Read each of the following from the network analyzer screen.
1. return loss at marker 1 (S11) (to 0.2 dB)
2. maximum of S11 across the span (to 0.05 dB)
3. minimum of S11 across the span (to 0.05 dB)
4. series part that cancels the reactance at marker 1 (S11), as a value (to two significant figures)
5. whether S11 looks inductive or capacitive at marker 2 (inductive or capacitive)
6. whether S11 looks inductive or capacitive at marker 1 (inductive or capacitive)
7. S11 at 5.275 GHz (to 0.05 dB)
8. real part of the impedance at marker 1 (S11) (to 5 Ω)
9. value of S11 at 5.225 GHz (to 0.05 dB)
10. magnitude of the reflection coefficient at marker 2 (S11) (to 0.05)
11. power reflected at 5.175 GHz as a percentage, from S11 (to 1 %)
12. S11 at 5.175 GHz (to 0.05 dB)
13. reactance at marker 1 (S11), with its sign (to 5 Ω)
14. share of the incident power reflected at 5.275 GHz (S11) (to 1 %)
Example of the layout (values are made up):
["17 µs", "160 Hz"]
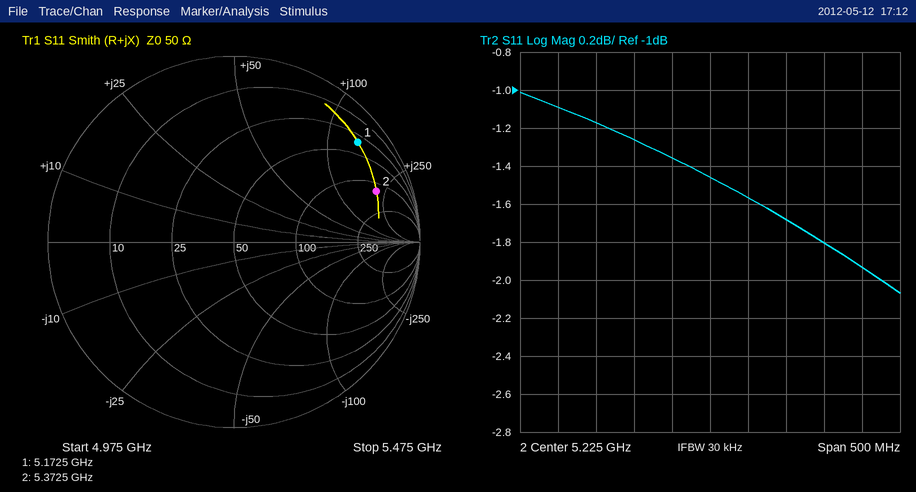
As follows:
["1.4 dB", "-1.00 dB", "-2.05 dB", "230 fF", "inductive", "inductive", "-1.55 dB", "35 Ω", "-1.45 dB", "0.80", "73 %", "-1.35 dB", "+135 Ω", "70 %"]
